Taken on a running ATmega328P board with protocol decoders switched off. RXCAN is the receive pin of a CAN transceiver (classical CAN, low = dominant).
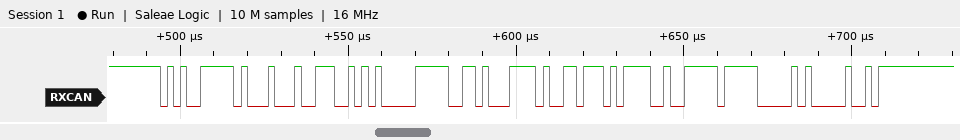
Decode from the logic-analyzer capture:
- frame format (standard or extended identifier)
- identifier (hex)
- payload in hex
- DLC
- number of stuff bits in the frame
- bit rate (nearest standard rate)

standard
0x53F
9C A8 3D A3 D3 75 E4 FF
8
7
500 kbit/s
